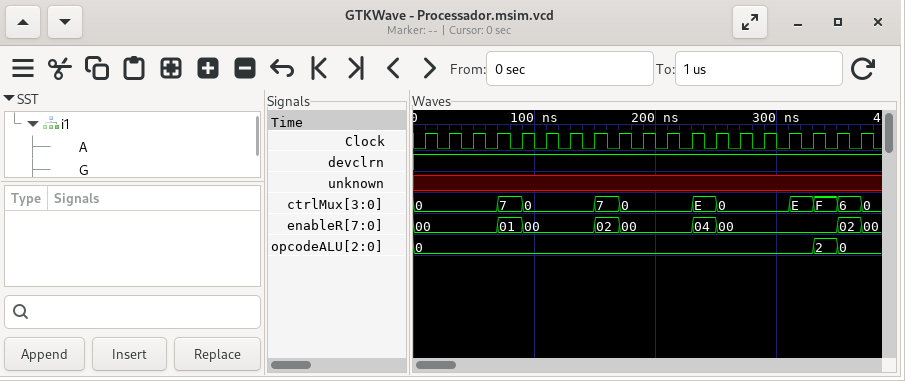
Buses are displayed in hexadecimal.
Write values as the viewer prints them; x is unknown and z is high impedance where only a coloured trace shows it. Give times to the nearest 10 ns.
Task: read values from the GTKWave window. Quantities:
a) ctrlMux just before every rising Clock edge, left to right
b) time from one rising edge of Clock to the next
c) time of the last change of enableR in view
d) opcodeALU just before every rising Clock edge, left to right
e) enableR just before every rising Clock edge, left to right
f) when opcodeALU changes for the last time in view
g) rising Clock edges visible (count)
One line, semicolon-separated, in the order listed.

0, 0, 0, 0, 7, 0, 0, 0, 7, 0, 0, 0, E, 0, 0, 0, E, F, 6; 20 ns; 370 ns; 0, 0, 0, 0, 0, 0, 0, 0, 0, 0, 0, 0, 0, 0, 0, 0, 0, 2, 0; 00, 00, 00, 00, 01, 00, 00, 00, 02, 00, 00, 00, 04, 00, 00, 00, 00, 00, 02; 350 ns; 19
